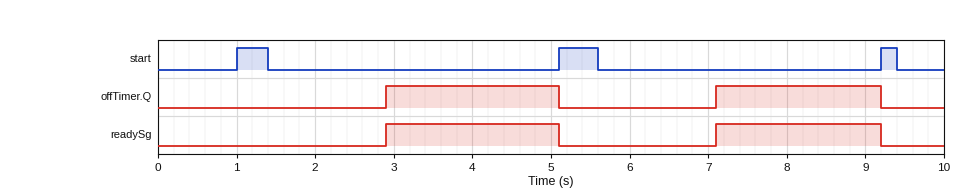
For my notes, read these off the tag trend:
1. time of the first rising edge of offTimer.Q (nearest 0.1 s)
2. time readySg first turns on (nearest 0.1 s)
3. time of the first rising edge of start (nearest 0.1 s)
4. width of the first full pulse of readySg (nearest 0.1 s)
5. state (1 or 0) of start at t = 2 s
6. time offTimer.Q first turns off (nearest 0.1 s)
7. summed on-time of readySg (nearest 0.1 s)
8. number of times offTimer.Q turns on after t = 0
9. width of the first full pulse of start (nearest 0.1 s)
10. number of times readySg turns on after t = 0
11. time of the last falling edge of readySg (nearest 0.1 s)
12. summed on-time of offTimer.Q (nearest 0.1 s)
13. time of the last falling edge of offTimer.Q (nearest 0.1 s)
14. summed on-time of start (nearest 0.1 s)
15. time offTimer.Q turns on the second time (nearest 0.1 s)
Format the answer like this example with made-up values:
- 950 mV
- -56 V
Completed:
- 2.9 s
- 2.9 s
- 1.0 s
- 2.2 s
- 0
- 5.1 s
- 4.3 s
- 2
- 0.4 s
- 2
- 9.2 s
- 4.3 s
- 9.2 s
- 1.1 s
- 7.1 s
